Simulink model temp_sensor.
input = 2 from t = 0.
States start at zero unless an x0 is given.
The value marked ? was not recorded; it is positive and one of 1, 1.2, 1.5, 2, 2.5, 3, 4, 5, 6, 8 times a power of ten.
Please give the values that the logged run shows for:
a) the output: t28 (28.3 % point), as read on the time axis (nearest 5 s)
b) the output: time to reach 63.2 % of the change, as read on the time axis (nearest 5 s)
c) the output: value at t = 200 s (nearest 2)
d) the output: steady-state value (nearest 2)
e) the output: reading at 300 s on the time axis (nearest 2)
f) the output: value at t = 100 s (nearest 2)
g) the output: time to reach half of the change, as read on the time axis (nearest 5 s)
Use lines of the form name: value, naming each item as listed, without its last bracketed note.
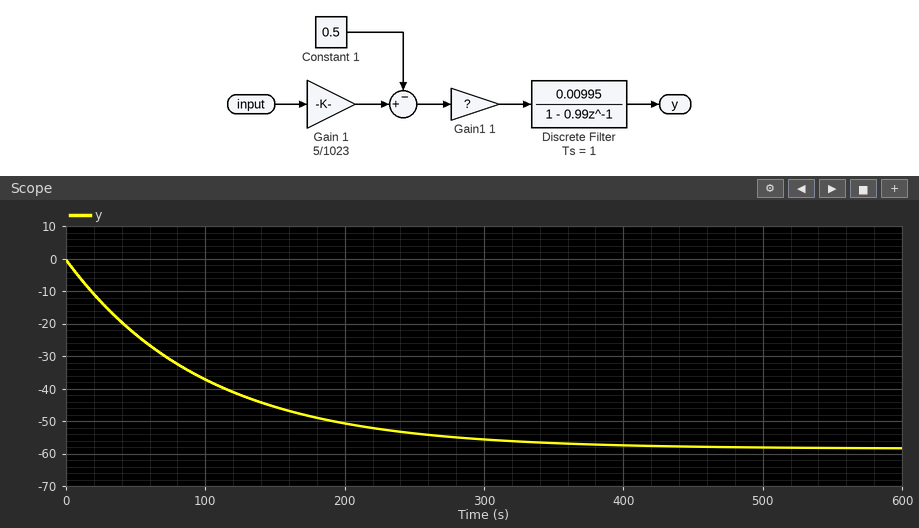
the output: t28 (28.3 % point), as read on the time axis: 35 s
the output: time to reach 63.2 % of the change, as read on the time axis: 100 s
the output: value at t = 200 s: -50
the output: steady-state value: -58
the output: reading at 300 s on the time axis: -56
the output: value at t = 100 s: -38
the output: time to reach half of the change, as read on the time axis: 70 s
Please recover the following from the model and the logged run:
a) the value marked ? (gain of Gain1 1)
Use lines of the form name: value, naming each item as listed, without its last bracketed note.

the value marked ?: 120
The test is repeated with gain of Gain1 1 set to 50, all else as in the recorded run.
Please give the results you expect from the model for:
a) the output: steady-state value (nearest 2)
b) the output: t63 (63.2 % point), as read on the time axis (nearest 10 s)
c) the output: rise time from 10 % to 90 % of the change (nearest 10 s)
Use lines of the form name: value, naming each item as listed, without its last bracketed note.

the output: steady-state value: -24
the output: t63 (63.2 % point), as read on the time axis: 100 s
the output: rise time from 10 % to 90 % of the change: 220 s
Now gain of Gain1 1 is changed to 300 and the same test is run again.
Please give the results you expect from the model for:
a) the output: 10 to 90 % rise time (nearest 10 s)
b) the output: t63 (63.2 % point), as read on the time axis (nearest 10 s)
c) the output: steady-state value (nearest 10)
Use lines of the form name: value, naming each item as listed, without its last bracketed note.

the output: 10 to 90 % rise time: 220 s
the output: t63 (63.2 % point), as read on the time axis: 100 s
the output: steady-state value: -150
